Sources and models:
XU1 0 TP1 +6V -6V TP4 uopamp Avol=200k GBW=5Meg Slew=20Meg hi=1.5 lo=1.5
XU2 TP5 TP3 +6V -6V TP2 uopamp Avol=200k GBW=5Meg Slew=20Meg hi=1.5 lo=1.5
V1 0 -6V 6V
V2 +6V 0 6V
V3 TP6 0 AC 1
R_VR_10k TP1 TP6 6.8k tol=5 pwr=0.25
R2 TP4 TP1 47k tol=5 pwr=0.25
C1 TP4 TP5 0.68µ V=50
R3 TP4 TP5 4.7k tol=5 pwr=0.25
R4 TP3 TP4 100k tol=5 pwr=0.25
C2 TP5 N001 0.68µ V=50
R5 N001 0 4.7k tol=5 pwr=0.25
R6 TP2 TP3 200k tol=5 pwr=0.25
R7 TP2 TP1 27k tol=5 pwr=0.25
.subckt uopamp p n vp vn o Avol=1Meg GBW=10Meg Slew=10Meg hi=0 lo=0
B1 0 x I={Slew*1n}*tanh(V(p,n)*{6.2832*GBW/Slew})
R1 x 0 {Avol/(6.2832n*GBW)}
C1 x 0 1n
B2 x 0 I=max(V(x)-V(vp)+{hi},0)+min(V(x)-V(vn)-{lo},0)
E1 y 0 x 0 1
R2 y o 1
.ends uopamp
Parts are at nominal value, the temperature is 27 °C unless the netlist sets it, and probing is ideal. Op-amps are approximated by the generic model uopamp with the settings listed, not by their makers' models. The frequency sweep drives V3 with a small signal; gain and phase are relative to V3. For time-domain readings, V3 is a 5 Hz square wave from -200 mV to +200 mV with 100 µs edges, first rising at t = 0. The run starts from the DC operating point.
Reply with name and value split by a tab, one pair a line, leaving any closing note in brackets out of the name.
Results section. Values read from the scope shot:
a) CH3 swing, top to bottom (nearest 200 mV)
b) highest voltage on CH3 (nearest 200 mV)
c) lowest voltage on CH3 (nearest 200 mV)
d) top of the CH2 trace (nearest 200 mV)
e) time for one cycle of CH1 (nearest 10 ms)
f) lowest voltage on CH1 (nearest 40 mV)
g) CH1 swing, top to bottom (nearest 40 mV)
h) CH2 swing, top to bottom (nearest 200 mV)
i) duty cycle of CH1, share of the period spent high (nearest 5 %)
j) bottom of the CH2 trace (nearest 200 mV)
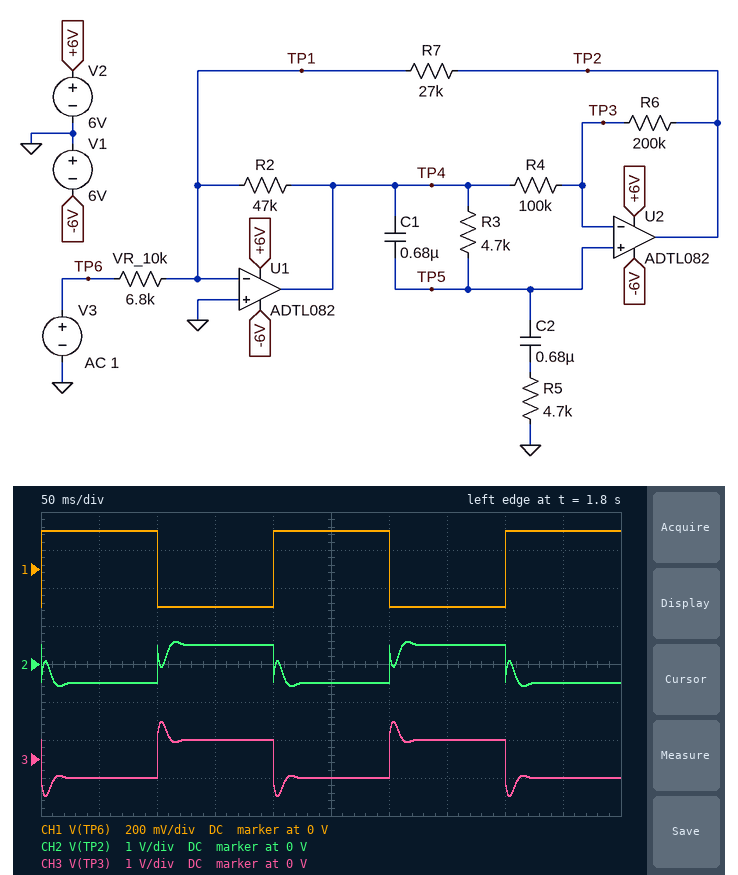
CH3 swing, top to bottom	2.0 V
highest voltage on CH3	1.0 V
lowest voltage on CH3	-1.0 V
top of the CH2 trace	600 mV
time for one cycle of CH1	200 ms
lowest voltage on CH1	-200 mV
CH1 swing, top to bottom	400 mV
CH2 swing, top to bottom	1.2 V
duty cycle of CH1, share of the period spent high	50 %
bottom of the CH2 trace	-600 mV
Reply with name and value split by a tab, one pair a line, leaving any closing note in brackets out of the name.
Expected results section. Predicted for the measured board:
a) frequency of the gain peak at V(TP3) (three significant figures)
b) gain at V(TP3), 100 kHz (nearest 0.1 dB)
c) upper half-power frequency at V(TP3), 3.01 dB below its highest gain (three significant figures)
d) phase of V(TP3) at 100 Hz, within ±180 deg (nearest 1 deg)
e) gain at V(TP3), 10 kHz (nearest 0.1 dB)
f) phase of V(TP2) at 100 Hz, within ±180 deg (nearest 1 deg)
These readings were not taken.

frequency of the gain peak at V(TP3)	49.8 Hz
gain at V(TP3), 100 kHz	8.0 dB
upper half-power frequency at V(TP3), 3.01 dB below its highest gain	109 Hz
phase of V(TP3) at 100 Hz, within ±180 deg	163 deg
gain at V(TP3), 10 kHz	8.0 dB
phase of V(TP2) at 100 Hz, within ±180 deg	-144 deg
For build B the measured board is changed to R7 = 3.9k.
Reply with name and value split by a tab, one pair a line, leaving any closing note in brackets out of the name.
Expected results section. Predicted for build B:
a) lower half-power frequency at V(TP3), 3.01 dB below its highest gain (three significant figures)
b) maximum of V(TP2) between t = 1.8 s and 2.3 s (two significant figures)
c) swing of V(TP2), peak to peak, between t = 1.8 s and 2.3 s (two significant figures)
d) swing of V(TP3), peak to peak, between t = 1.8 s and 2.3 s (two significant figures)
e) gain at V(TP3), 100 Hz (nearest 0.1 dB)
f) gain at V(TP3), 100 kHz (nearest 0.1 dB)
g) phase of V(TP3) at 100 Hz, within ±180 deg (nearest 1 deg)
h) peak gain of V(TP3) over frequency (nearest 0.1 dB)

lower half-power frequency at V(TP3), 3.01 dB below its highest gain	44.3 Hz
maximum of V(TP2) between t = 1.8 s and 2.3 s	130 mV
swing of V(TP2), peak to peak, between t = 1.8 s and 2.3 s	270 mV
swing of V(TP3), peak to peak, between t = 1.8 s and 2.3 s	830 mV
gain at V(TP3), 100 Hz	-1.2 dB
gain at V(TP3), 100 kHz	-5.5 dB
phase of V(TP3) at 100 Hz, within ±180 deg	136 deg
peak gain of V(TP3) over frequency	13.3 dB
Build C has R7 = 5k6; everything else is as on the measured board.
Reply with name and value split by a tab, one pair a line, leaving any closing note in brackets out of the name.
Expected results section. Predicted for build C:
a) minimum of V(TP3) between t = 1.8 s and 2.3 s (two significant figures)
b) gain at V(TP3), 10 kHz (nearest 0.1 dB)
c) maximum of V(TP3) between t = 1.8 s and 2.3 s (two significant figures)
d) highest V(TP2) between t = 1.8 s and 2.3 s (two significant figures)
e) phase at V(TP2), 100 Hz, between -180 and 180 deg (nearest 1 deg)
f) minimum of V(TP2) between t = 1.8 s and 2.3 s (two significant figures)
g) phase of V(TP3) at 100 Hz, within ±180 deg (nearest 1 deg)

minimum of V(TP3) between t = 1.8 s and 2.3 s	-540 mV
gain at V(TP3), 10 kHz	-2.7 dB
maximum of V(TP3) between t = 1.8 s and 2.3 s	540 mV
highest V(TP2) between t = 1.8 s and 2.3 s	190 mV
phase at V(TP2), 100 Hz, between -180 and 180 deg	-168 deg
minimum of V(TP2) between t = 1.8 s and 2.3 s	-190 mV
phase of V(TP3) at 100 Hz, within ±180 deg	139 deg
